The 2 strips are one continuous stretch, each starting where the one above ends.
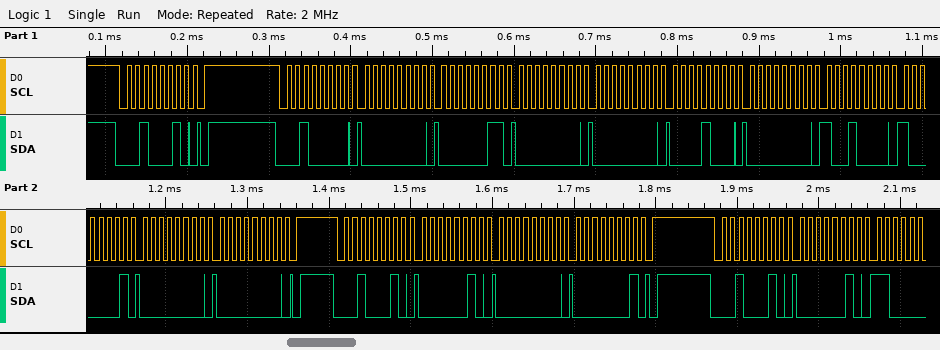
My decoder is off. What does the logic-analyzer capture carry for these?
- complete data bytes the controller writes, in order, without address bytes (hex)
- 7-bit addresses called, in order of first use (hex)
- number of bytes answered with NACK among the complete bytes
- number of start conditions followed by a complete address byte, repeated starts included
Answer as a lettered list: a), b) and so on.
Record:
a) 00 03 00 00 08 00 90 81 00 00 02 00 01 02
b) 0x11 0x10
c) 0
d) 4
